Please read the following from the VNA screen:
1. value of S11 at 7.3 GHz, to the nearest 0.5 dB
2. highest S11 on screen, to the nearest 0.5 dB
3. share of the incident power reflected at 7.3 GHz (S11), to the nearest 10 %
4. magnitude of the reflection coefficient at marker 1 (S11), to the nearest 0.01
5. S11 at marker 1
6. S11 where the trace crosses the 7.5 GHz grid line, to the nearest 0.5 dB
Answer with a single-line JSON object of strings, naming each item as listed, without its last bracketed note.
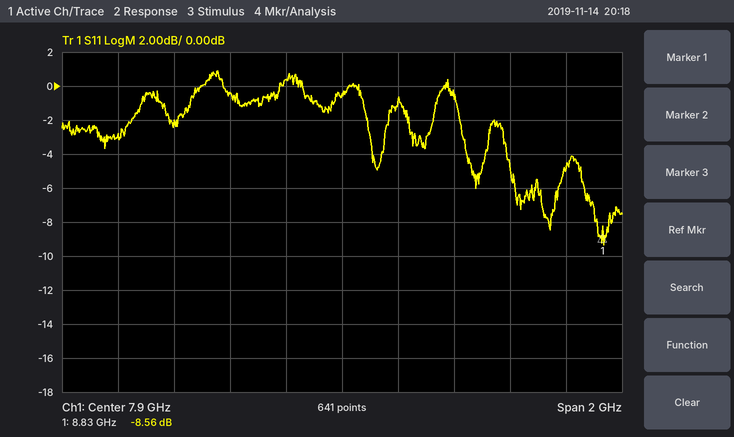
{"value of S11 at 7.3 GHz, to the nearest 0.5 dB": "-2.0 dB", "highest S11 on screen, to the nearest 0.5 dB": "1.0 dB", "share of the incident power reflected at 7.3 GHz (S11), to the nearest 10 %": "60 %", "magnitude of the reflection coefficient at marker 1 (S11), to the nearest 0.01": "0.37", "S11 at marker 1": "-8.56 dB", "S11 where the trace crosses the 7.5 GHz grid line, to the nearest 0.5 dB": "-0.5 dB"}
